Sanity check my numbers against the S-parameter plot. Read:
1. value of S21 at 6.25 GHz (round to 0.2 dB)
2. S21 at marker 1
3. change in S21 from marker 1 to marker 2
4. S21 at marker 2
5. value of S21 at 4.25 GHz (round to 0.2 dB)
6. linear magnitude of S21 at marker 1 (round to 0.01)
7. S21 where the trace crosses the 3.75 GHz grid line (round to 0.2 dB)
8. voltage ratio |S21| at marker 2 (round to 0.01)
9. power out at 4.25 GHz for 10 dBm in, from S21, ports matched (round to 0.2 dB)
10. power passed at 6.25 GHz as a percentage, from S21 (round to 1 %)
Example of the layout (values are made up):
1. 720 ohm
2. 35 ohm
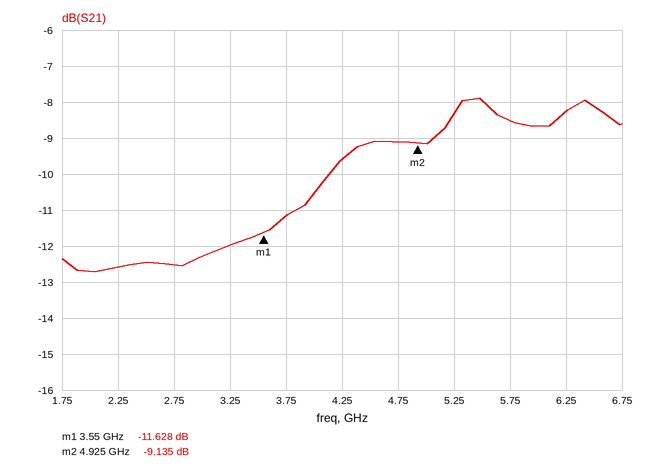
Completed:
1. -8.2 dB
2. -11.628 dB
3. 2.493 dB
4. -9.135 dB
5. -9.6 dB
6. 0.26
7. -11.2 dB
8. 0.35
9. 0.4 dBm
10. 15 %
